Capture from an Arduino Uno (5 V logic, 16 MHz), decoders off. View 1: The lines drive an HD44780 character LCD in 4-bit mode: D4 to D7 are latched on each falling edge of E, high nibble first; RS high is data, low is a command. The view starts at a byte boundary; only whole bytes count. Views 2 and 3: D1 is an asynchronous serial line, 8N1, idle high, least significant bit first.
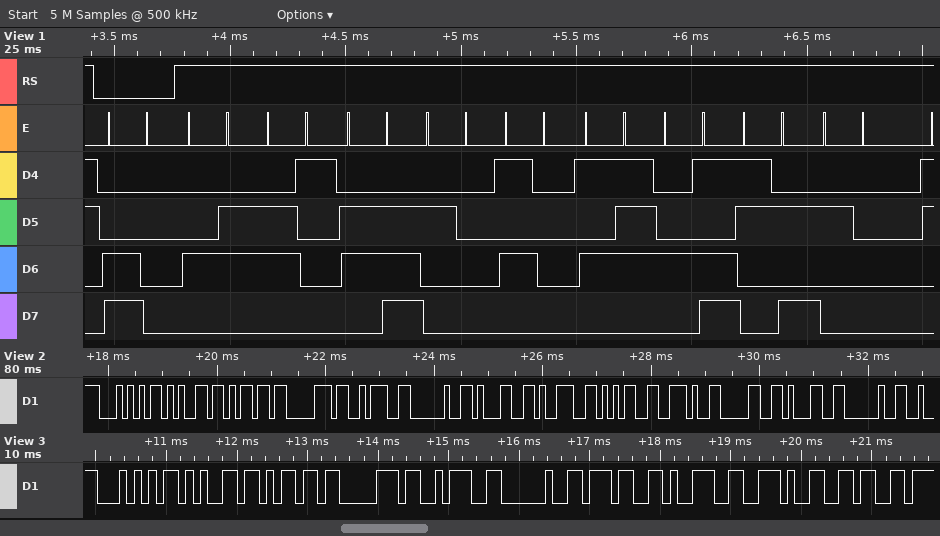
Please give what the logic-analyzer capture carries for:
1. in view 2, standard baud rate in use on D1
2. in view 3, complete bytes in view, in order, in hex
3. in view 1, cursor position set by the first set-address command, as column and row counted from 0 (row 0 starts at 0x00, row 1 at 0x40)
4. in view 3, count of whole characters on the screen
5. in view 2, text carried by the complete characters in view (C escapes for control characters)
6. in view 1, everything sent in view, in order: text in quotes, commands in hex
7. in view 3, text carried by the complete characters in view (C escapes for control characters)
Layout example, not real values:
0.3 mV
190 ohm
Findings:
9600 baud
0x54 0x65 0x6D 0x70 0x3A 0x20 0x37 0x39 0x2E 0x36
column 0, row 1
10
"Temp: 195.01 "
0xC0 "Fan PWM: "
"Temp: 79.6"
